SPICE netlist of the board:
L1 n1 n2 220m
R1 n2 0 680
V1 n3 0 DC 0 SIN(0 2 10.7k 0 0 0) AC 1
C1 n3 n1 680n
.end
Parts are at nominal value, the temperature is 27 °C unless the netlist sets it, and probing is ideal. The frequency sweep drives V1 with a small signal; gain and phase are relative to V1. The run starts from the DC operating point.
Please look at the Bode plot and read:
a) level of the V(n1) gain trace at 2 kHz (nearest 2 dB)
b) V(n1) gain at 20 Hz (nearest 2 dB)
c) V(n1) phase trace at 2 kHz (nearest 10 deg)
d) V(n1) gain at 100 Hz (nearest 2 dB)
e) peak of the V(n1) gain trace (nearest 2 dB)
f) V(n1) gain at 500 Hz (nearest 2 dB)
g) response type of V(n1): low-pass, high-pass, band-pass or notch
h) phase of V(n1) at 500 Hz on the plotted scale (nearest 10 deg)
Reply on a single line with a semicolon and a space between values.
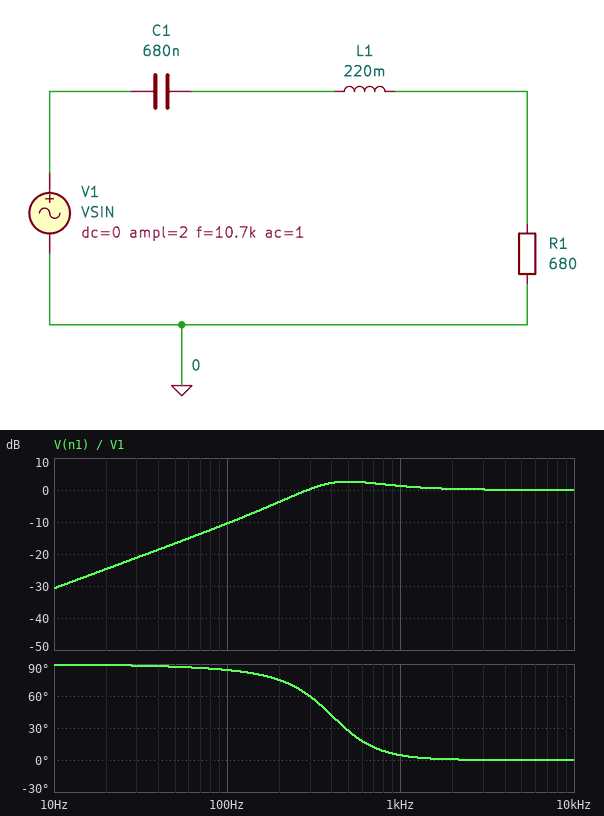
0 dB; -24 dB; 0 deg; -10 dB; 2 dB; 2 dB; high-pass; 30 deg
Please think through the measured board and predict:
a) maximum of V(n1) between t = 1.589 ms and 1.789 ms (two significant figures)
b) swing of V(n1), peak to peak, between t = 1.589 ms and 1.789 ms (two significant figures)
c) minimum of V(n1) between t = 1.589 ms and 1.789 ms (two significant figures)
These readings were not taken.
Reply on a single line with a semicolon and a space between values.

2.0 V; 4.0 V; -2.0 V
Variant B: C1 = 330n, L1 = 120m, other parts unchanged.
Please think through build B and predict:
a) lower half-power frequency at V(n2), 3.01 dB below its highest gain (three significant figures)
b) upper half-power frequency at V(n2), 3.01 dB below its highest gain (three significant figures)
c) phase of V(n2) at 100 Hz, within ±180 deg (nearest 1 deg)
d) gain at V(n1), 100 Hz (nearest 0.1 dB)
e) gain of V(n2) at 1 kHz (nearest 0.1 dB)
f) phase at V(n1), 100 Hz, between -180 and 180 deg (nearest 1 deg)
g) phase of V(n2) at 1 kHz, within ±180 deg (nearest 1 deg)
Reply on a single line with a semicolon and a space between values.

467 Hz; 1.37 kHz; 82 deg; -16.9 dB; -0.6 dB; 88 deg; -22 deg
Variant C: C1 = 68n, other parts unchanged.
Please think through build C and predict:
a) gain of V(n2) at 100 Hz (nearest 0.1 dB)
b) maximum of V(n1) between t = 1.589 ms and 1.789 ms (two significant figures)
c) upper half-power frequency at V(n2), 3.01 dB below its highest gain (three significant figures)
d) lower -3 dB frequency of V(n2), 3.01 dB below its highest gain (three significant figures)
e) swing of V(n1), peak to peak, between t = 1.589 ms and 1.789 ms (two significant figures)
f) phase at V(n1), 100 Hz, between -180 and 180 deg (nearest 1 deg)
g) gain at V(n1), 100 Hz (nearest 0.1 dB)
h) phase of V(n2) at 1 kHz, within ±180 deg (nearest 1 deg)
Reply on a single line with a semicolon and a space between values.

-30.7 dB; 2.0 V; 1.57 kHz; 1.08 kHz; 4.1 V; 100 deg; -30.5 dB; 55 deg
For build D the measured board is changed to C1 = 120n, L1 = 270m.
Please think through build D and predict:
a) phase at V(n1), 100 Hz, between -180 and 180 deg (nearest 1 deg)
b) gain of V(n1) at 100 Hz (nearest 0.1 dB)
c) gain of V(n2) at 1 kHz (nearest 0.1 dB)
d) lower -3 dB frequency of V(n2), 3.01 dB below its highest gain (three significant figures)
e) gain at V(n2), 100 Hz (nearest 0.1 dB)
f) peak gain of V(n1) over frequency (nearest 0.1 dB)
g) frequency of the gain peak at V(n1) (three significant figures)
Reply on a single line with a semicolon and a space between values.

101 deg; -25.4 dB; -1.1 dB; 706 Hz; -25.7 dB; 7.8 dB; 925 Hz
